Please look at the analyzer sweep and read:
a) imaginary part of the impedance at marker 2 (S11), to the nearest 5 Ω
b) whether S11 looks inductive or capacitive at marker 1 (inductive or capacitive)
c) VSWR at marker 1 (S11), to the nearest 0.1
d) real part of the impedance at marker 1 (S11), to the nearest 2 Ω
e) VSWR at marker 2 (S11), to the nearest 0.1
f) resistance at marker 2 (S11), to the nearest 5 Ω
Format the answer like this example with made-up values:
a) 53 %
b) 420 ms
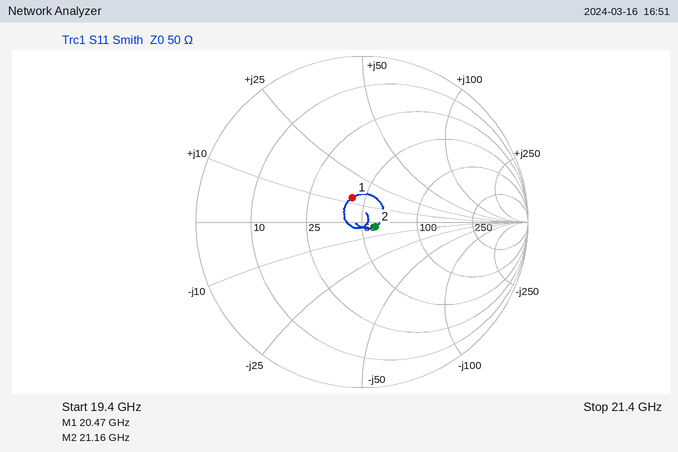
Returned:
a) -5 Ω
b) inductive
c) 1.4
d) 42 Ω
e) 1.2
f) 60 Ω
